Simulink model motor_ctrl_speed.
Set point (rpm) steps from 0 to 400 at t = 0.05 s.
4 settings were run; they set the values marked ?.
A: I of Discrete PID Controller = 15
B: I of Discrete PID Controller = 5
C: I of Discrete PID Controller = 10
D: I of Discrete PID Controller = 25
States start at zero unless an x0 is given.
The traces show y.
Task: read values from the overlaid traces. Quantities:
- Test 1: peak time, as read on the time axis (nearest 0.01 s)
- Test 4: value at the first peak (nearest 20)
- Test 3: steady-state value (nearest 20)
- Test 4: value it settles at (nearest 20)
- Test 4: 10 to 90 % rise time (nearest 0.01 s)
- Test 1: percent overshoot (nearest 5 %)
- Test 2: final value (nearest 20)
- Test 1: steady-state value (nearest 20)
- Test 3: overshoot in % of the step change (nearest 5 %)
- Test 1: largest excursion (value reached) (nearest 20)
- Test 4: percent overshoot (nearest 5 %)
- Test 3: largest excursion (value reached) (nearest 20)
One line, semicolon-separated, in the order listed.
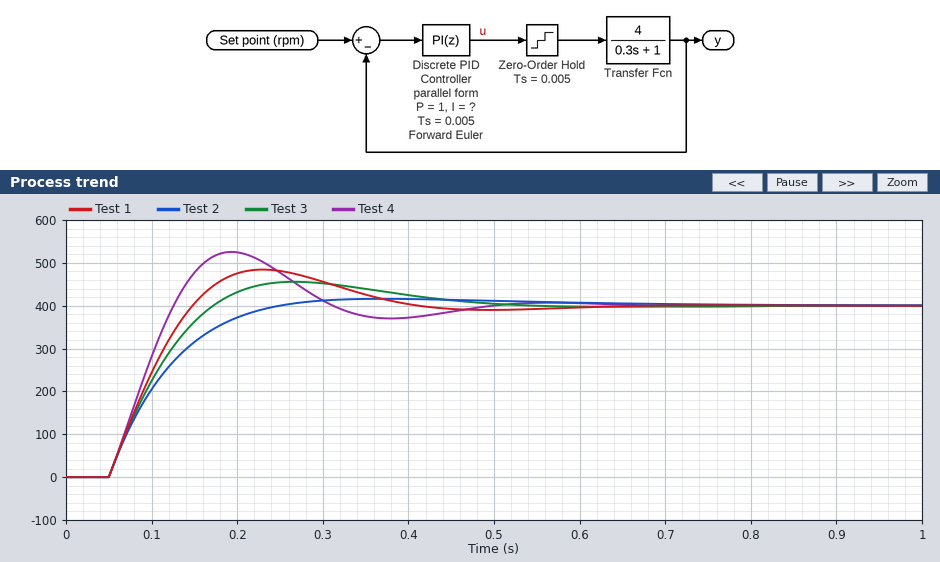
0.23 s; 520; 400; 400; 0.06 s; 20 %; 400; 400; 15 %; 480; 30 %; 460
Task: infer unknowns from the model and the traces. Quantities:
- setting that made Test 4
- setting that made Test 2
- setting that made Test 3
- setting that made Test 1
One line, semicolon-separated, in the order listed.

D; B; C; A
